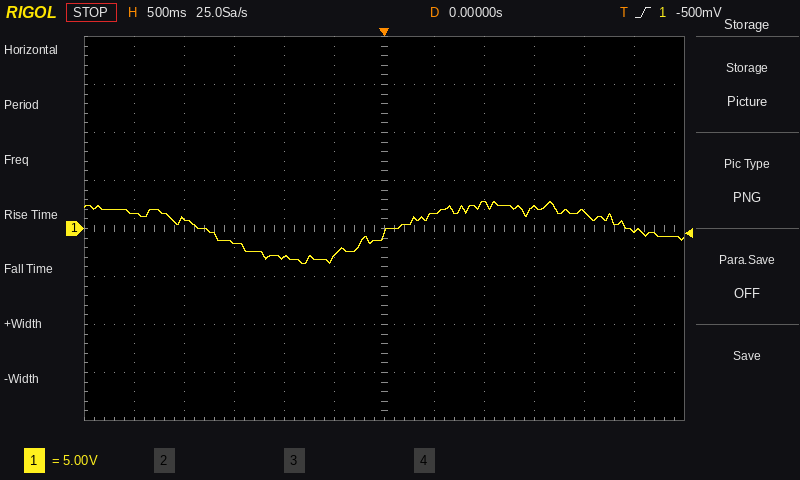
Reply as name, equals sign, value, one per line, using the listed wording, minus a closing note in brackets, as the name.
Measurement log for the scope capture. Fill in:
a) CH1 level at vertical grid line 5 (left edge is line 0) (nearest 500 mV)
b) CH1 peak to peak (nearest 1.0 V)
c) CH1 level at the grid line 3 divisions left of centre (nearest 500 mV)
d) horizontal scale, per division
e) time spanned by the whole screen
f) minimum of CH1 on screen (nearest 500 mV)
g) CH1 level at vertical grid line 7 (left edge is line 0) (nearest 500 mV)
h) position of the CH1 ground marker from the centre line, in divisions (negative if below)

CH1 level at vertical grid line 5 (left edge is line 0) = -3.0 V
CH1 peak to peak = 6.0 V
CH1 level at the grid line 3 divisions left of centre = -1.5 V
horizontal scale, per division = 500 ms
time spanned by the whole screen = 6 s
minimum of CH1 on screen = -3.5 V
CH1 level at vertical grid line 7 (left edge is line 0) = 1.5 V
position of the CH1 ground marker from the centre line, in divisions = 0.0 div
